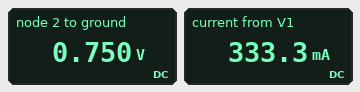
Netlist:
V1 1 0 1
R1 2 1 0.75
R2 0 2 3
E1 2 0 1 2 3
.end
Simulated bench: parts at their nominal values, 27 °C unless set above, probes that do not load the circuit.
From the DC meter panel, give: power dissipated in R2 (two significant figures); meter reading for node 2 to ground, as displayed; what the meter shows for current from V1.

190 mW
0.750 V
333.3 mA
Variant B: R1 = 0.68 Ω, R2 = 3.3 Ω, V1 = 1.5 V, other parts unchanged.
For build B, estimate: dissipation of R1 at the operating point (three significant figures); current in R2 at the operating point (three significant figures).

207 mW
341 mA
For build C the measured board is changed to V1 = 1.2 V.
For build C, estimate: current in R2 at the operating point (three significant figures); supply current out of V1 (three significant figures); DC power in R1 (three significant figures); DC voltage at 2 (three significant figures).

300 mA
400 mA
120 mW
900 mV
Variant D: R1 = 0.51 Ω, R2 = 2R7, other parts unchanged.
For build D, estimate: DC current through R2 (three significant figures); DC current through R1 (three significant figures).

278 mA
490 mA
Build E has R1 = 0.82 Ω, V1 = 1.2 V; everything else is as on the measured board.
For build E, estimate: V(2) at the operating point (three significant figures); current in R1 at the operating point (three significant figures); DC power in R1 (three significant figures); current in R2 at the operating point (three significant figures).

900 mV
366 mA
110 mW
300 mA
